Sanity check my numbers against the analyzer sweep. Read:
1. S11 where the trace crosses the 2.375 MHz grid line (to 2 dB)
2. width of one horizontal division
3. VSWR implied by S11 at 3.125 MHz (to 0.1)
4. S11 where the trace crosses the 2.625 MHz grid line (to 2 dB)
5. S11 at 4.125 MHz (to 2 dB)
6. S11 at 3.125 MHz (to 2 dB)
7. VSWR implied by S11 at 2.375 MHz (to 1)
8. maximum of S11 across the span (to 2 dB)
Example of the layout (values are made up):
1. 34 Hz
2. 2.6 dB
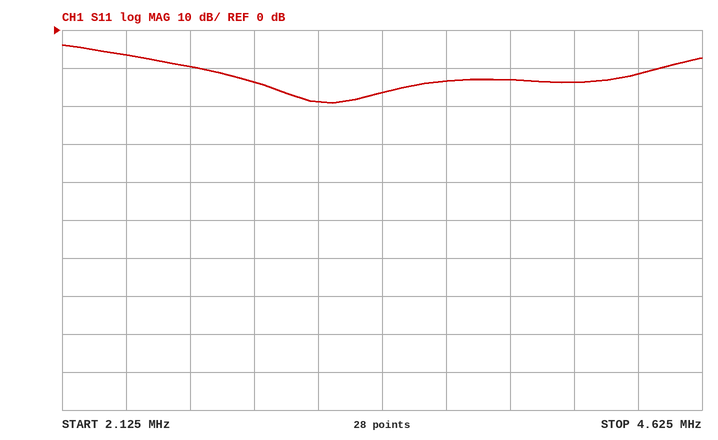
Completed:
1. -6 dB
2. 250 kHz
3. 1.3
4. -10 dB
5. -14 dB
6. -18 dB
7. 3
8. -4 dB
